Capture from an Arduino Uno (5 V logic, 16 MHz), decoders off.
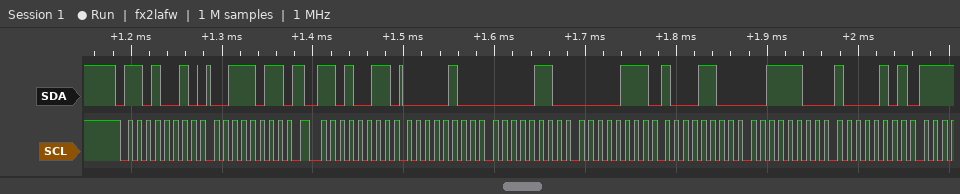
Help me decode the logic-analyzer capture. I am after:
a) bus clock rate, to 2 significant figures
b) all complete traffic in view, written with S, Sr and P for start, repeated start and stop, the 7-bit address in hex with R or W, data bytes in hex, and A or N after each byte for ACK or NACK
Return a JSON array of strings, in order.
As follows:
["100 kHz", "S 69W A 3B A Sr 69R A 04 A 06 A 07 A 8C A 3C A 85 A"]
